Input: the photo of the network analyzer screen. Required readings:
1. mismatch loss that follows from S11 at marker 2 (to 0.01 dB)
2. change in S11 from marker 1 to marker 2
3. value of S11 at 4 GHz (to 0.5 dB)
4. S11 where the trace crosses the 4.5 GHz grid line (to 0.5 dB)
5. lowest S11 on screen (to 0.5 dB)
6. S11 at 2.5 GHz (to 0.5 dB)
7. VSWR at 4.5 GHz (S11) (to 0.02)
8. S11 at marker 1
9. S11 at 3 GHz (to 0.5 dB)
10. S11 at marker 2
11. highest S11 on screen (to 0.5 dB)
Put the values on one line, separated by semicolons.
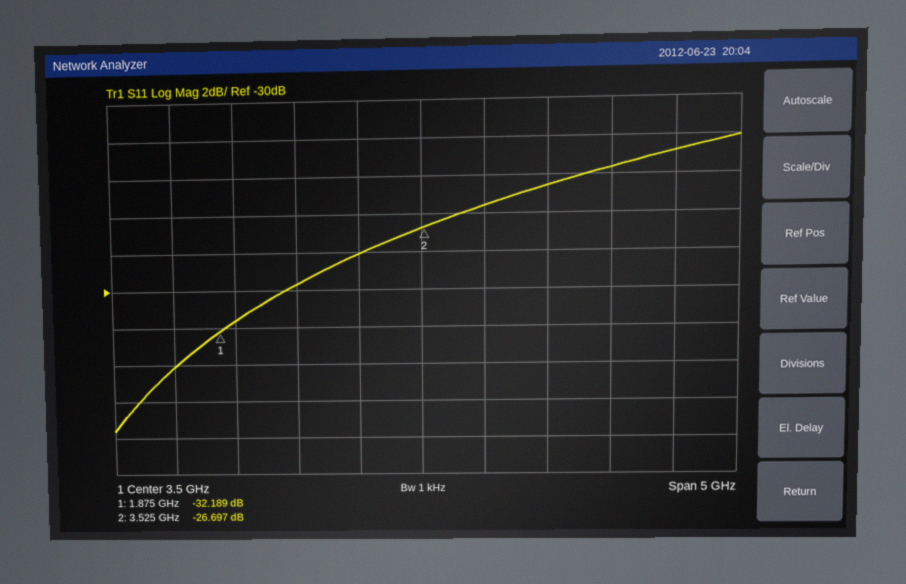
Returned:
0.01 dB; 5.492 dB; -25.5 dB; -24.5 dB; -37.5 dB; -29.5 dB; 1.12; -32.189 dB; -28.0 dB; -26.697 dB; -22.0 dB
